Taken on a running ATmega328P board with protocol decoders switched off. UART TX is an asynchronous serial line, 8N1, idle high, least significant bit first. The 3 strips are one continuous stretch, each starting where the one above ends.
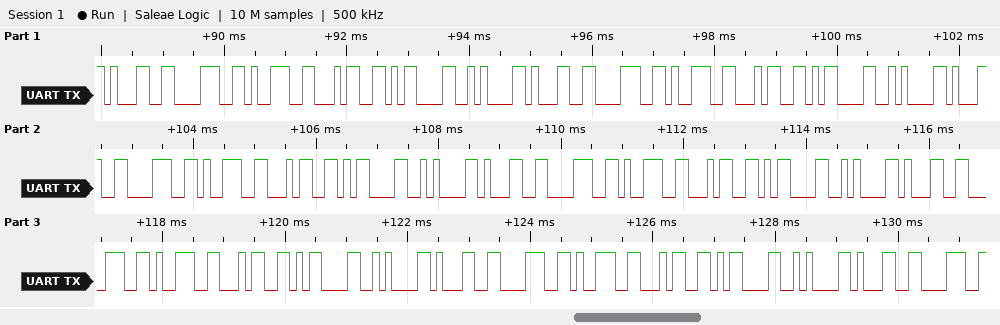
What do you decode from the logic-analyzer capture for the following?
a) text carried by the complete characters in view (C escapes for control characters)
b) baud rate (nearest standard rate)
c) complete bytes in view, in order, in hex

"1894\r\n1894\r\n1894\r\n1894\r\n1894\r\n1894\r\n18"
9600 baud
31 38 39 34 0D 0A 31 38 39 34 0D 0A 31 38 39 34 0D 0A 31 38 39 34 0D 0A 31 38 39 34 0D 0A 31 38 39 34 0D 0A 31 38
